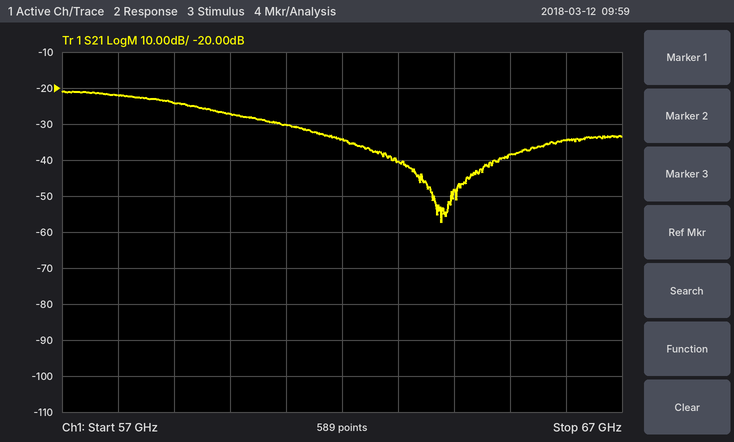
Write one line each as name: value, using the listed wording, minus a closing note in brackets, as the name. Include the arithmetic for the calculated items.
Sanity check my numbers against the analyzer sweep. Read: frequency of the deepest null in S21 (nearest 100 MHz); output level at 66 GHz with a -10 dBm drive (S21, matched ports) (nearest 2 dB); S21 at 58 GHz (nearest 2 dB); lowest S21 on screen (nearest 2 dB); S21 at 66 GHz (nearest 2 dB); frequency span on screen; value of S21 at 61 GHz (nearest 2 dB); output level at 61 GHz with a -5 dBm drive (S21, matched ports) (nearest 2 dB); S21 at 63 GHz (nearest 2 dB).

frequency of the deepest null in S21: 63.8 GHz
output level at 66 GHz with a -10 dBm drive (S21, matched ports): -10 dBm + (-34 dB) = -44 dBm
S21 at 58 GHz: -22 dB
lowest S21 on screen: -58 dB
S21 at 66 GHz: -34 dB
frequency span on screen: 10 GHz
value of S21 at 61 GHz: -30 dB
output level at 61 GHz with a -5 dBm drive (S21, matched ports): -5 dBm + (-30 dB) = -36 dBm
S21 at 63 GHz: -40 dB
